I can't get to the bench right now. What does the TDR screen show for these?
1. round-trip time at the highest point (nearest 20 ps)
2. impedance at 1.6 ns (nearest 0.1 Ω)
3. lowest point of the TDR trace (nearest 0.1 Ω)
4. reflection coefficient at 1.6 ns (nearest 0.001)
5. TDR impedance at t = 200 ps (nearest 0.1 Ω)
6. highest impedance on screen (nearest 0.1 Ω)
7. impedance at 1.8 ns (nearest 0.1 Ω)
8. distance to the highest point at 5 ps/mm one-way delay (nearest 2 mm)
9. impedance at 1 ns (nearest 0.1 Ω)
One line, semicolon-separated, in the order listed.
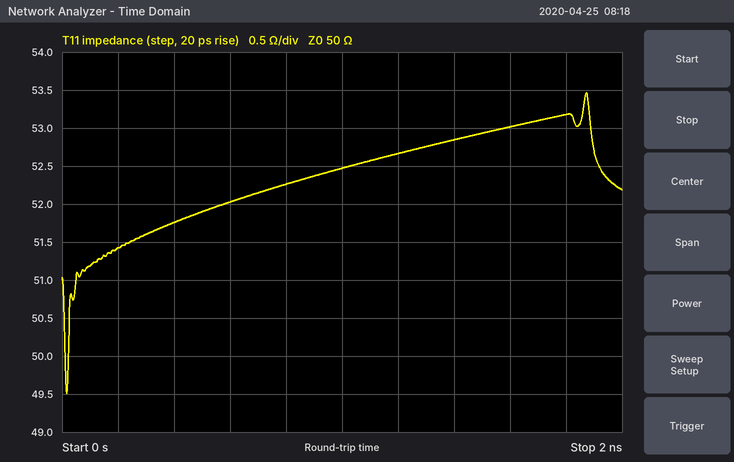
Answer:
1.88 ns; 53.0 Ω; 49.5 Ω; +0.029; 51.4 Ω; 53.5 Ω; 53.2 Ω; 188 mm; 52.5 Ω
